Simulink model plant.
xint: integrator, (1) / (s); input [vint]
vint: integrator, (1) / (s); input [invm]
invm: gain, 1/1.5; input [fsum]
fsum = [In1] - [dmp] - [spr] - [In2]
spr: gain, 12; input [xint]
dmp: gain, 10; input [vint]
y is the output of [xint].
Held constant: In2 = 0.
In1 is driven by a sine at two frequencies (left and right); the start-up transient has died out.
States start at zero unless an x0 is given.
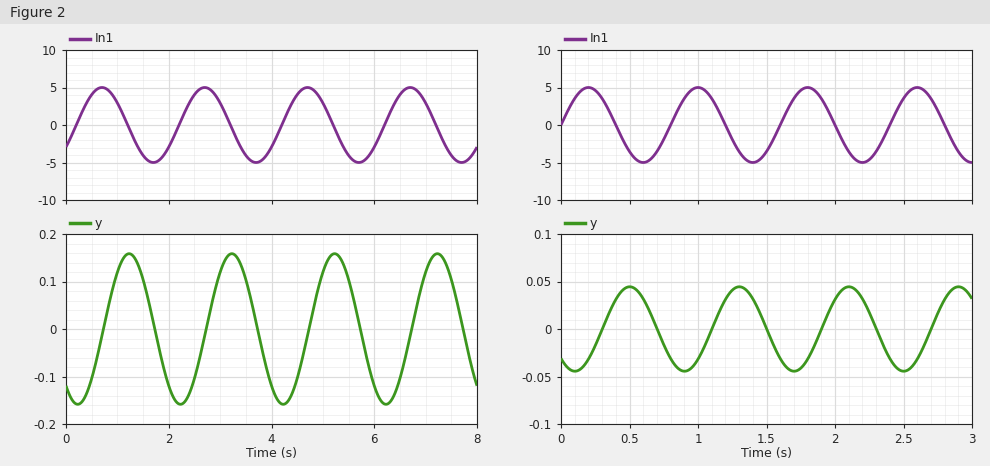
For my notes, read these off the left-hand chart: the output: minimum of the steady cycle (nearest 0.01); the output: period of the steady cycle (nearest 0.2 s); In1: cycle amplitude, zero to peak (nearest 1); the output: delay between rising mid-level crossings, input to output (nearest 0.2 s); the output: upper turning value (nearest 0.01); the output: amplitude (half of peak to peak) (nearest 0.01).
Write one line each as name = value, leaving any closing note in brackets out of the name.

the output: minimum of the steady cycle = -0.16
the output: period of the steady cycle = 2.0 s
In1: cycle amplitude, zero to peak = 5
the output: delay between rising mid-level crossings, input to output = 0.6 s
the output: upper turning value = 0.16
the output: amplitude (half of peak to peak) = 0.16
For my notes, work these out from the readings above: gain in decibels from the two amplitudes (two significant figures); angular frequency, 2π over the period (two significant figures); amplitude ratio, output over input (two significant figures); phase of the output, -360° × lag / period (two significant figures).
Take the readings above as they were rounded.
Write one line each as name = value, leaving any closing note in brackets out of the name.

gain in decibels from the two amplitudes = -30 dB
angular frequency, 2π over the period = 3.1 rad/s
amplitude ratio, output over input = 0.032
phase of the output, -360° × lag / period = -110°
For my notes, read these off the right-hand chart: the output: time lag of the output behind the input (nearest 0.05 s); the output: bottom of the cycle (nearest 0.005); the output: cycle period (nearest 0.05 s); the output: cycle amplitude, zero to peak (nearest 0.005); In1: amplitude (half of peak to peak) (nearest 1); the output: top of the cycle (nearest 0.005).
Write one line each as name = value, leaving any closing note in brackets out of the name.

the output: time lag of the output behind the input = 0.30 s
the output: bottom of the cycle = -0.045
the output: cycle period = 0.80 s
the output: cycle amplitude, zero to peak = 0.045
In1: amplitude (half of peak to peak) = 5
the output: top of the cycle = 0.045
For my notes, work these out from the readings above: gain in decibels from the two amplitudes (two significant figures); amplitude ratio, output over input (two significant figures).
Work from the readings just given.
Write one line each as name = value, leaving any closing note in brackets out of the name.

gain in decibels from the two amplitudes = -41 dB
amplitude ratio, output over input = 0.0090
